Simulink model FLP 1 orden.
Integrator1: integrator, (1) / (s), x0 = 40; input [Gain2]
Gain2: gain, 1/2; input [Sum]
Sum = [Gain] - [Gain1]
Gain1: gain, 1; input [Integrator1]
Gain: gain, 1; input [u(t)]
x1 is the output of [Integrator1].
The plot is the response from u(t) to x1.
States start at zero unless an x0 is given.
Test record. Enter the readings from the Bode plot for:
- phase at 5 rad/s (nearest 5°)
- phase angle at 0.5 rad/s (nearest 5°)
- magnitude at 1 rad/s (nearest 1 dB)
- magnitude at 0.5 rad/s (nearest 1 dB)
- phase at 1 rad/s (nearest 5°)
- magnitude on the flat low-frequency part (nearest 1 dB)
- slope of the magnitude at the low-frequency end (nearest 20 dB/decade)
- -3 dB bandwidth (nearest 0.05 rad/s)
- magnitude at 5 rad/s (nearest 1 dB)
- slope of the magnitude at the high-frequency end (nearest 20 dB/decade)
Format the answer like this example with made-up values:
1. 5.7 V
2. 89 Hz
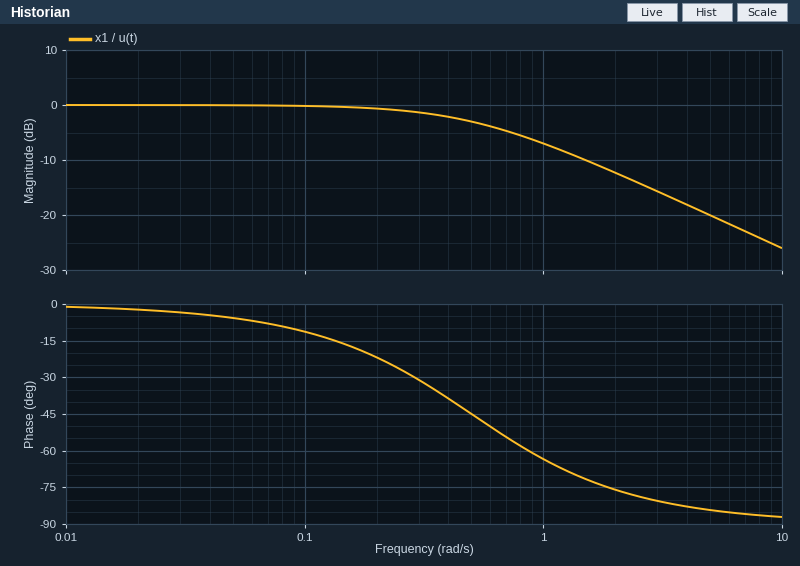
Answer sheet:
1. -85°
2. -45°
3. -7 dB
4. -3 dB
5. -65°
6. 0 dB
7. 0 dB/decade
8. 0.50 rad/s
9. -20 dB
10. -20 dB/decade
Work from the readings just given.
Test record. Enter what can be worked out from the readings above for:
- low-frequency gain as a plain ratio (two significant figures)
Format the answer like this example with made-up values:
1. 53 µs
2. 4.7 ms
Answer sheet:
1. 1.0
